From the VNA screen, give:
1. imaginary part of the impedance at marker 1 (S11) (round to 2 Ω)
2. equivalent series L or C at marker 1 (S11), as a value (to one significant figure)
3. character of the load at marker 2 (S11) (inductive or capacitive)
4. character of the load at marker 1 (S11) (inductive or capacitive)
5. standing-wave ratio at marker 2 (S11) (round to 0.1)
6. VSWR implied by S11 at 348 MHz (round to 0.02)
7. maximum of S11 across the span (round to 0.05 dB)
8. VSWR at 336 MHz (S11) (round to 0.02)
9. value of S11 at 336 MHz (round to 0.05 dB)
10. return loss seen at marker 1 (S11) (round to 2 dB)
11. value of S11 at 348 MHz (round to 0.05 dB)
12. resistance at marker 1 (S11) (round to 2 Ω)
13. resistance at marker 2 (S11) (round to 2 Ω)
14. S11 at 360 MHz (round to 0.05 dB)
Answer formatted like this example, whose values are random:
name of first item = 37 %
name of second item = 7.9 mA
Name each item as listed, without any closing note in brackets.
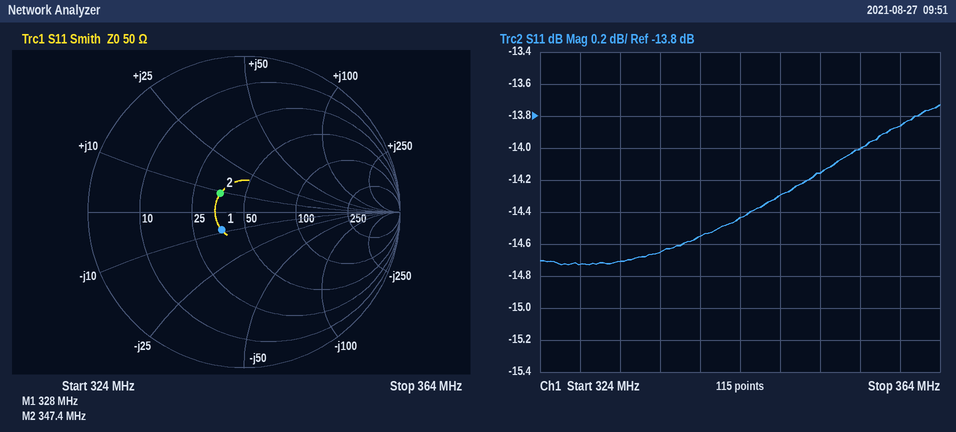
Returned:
imaginary part of the impedance at marker 1 (S11) = -8 Ω
equivalent series L or C at marker 1 (S11), as a value = 60 pF
character of the load at marker 2 (S11) = inductive
character of the load at marker 1 (S11) = capacitive
standing-wave ratio at marker 2 (S11) = 1.5
VSWR implied by S11 at 348 MHz = 1.48
maximum of S11 across the span = -13.75 dB
VSWR at 336 MHz (S11) = 1.46
value of S11 at 336 MHz = -14.65 dB
return loss seen at marker 1 (S11) = 14 dB
value of S11 at 348 MHz = -14.30 dB
resistance at marker 1 (S11) = 36 Ω
resistance at marker 2 (S11) = 36 Ω
S11 at 360 MHz = -13.85 dB
